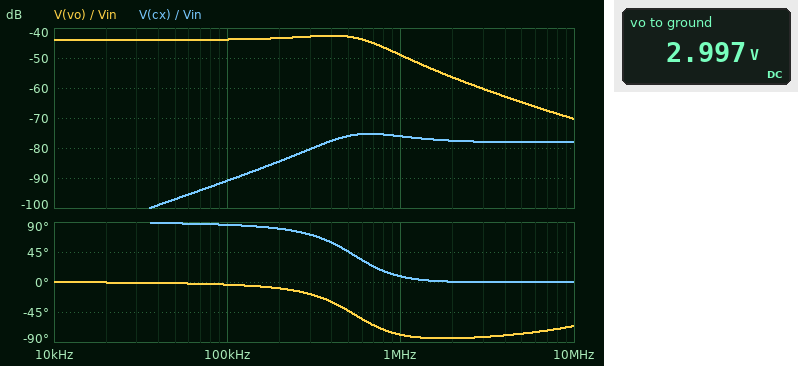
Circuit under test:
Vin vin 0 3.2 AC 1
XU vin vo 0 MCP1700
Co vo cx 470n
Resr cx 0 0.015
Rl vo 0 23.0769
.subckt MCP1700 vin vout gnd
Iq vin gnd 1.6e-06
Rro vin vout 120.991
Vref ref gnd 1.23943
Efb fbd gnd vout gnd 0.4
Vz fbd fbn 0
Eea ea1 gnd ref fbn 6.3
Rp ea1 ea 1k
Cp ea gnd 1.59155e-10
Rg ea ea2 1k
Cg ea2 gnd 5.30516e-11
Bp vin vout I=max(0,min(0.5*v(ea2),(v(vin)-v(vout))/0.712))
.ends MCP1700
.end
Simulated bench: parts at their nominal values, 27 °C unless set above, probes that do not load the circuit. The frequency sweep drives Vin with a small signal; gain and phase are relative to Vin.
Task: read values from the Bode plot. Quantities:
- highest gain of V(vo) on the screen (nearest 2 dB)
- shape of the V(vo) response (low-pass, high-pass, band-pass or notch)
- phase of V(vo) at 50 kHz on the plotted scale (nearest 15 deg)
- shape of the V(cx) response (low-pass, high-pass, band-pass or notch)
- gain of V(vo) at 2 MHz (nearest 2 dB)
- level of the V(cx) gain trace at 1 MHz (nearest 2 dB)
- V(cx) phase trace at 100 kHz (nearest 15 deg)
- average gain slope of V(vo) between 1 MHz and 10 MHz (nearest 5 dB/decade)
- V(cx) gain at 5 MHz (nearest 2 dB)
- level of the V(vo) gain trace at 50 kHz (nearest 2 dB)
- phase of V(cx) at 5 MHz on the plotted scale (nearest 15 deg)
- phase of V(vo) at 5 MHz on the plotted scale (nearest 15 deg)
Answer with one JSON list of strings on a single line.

["-42 dB", "low-pass", "0 deg", "high-pass", "-56 dB", "-76 dB", "90 deg", "-20 dB/decade", "-78 dB", "-44 dB", "0 deg", "-75 deg"]
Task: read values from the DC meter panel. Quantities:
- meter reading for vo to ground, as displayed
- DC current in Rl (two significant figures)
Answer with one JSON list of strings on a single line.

["2.997 V", "130 mA"]
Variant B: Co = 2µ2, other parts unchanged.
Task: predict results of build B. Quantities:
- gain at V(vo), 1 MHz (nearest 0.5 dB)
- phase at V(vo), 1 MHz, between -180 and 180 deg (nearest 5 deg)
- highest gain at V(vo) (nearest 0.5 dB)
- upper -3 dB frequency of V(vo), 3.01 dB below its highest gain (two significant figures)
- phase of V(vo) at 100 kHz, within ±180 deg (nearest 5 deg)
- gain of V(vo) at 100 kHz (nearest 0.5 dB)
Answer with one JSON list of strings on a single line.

["-64.0 dB", "-75 deg", "-44.0 dB", "110 kHz", "-40 deg", "-46.5 dB"]
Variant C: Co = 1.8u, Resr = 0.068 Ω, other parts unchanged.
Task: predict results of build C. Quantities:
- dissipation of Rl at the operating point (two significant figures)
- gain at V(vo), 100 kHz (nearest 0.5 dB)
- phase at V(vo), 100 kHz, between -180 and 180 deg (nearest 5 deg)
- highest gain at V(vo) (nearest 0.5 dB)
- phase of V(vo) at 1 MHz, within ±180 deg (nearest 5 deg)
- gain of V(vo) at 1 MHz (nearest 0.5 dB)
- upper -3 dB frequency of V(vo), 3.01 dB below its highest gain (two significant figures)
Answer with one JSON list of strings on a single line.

["390 mW", "-46.0 dB", "-35 deg", "-44.0 dB", "-50 deg", "-60.5 dB", "130 kHz"]
